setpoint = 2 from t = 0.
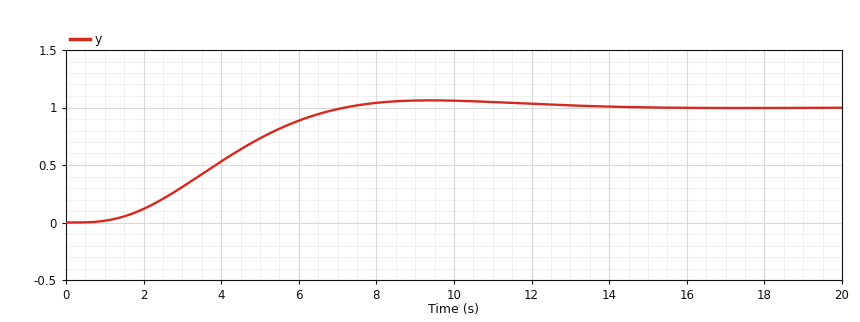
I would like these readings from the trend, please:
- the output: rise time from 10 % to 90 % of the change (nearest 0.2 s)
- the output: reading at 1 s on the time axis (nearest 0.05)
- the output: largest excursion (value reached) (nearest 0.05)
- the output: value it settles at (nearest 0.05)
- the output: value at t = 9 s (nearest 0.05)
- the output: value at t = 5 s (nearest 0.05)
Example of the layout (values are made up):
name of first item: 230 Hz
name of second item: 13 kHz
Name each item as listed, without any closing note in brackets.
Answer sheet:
the output: rise time from 10 % to 90 % of the change: 4.2 s
the output: reading at 1 s on the time axis: 0.00
the output: largest excursion (value reached): 1.05
the output: value it settles at: 1.00
the output: value at t = 9 s: 1.05
the output: value at t = 5 s: 0.75
